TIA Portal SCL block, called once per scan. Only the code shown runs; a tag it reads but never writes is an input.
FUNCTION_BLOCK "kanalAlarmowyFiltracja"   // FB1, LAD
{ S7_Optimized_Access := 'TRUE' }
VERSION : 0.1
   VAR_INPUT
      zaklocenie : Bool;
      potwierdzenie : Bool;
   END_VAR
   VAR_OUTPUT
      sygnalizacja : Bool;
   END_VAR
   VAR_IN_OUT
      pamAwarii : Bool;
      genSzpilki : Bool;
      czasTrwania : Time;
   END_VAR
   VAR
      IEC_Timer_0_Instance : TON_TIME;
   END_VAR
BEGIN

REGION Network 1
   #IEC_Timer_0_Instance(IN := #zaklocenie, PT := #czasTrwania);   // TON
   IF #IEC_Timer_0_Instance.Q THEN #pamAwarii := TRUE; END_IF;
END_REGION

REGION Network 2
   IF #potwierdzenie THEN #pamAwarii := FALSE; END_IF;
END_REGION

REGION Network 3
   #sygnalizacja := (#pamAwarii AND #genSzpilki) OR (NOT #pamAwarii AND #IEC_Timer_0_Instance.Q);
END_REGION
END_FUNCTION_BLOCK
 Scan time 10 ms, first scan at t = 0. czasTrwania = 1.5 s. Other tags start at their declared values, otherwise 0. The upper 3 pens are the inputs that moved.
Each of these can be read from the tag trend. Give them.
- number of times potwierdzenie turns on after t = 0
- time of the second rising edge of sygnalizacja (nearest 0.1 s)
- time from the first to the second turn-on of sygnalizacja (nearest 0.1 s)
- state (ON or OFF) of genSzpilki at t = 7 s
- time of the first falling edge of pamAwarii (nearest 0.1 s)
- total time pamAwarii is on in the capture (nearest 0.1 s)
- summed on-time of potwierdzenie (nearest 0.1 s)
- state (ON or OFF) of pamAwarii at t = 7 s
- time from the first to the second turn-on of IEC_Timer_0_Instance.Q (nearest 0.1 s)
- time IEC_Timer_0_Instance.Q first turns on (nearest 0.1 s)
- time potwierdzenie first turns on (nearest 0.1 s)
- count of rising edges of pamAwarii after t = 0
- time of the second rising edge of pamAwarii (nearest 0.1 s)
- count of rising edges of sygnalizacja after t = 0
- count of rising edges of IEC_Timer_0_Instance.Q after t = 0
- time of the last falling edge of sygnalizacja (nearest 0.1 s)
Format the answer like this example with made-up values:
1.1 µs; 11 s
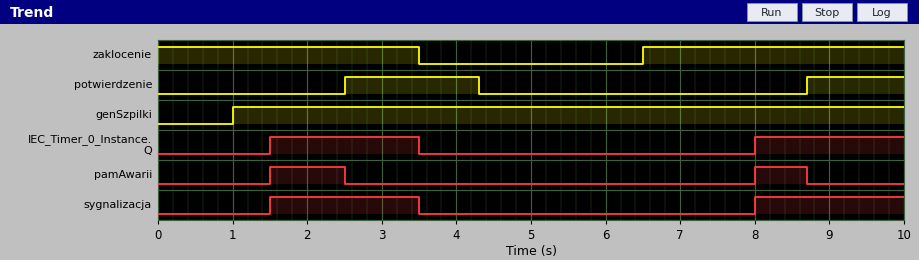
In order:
2; 8.0 s; 6.5 s; ON; 2.5 s; 1.7 s; 3.1 s; OFF; 6.5 s; 1.5 s; 2.5 s; 2; 8.0 s; 2; 2; 3.5 s
